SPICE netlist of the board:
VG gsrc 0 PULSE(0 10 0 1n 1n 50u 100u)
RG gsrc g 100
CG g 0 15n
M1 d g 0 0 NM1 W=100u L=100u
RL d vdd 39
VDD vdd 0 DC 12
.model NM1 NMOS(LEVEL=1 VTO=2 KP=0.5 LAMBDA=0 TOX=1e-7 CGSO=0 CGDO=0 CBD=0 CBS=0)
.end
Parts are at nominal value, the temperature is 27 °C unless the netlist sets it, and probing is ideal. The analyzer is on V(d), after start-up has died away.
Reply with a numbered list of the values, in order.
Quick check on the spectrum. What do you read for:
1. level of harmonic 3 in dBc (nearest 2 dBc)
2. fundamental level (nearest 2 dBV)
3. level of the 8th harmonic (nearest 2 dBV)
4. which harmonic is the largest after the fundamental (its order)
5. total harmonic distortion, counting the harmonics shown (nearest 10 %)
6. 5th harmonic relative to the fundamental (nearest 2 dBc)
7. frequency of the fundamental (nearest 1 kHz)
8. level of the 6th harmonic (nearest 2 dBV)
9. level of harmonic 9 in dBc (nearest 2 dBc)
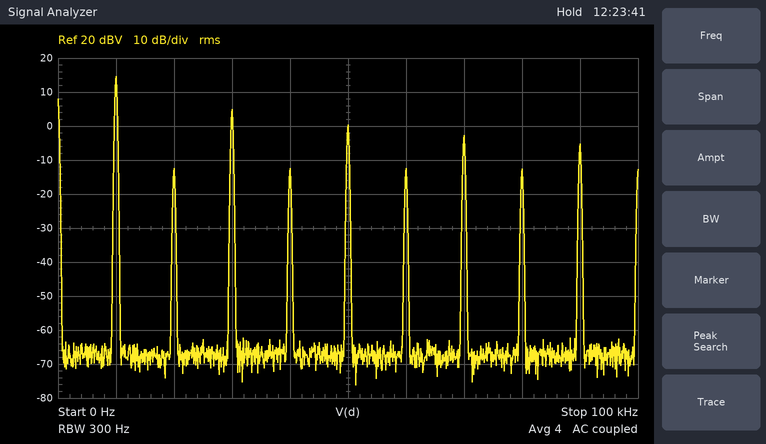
1. -10 dBc
2. 14 dBV
3. -12 dBV
4. 3
5. 40 %
6. -14 dBc
7. 10 kHz
8. -12 dBV
9. -20 dBc
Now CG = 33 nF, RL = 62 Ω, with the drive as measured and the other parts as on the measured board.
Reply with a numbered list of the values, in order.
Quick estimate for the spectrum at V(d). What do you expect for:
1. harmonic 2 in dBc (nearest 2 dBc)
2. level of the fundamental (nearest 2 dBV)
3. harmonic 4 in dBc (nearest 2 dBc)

1. -20 dBc
2. 14 dBV
3. -20 dBc
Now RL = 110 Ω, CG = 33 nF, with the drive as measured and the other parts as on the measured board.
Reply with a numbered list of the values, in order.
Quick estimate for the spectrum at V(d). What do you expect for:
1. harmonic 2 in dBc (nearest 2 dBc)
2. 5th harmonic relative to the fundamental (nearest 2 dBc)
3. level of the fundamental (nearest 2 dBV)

1. -18 dBc
2. -16 dBc
3. 14 dBV
